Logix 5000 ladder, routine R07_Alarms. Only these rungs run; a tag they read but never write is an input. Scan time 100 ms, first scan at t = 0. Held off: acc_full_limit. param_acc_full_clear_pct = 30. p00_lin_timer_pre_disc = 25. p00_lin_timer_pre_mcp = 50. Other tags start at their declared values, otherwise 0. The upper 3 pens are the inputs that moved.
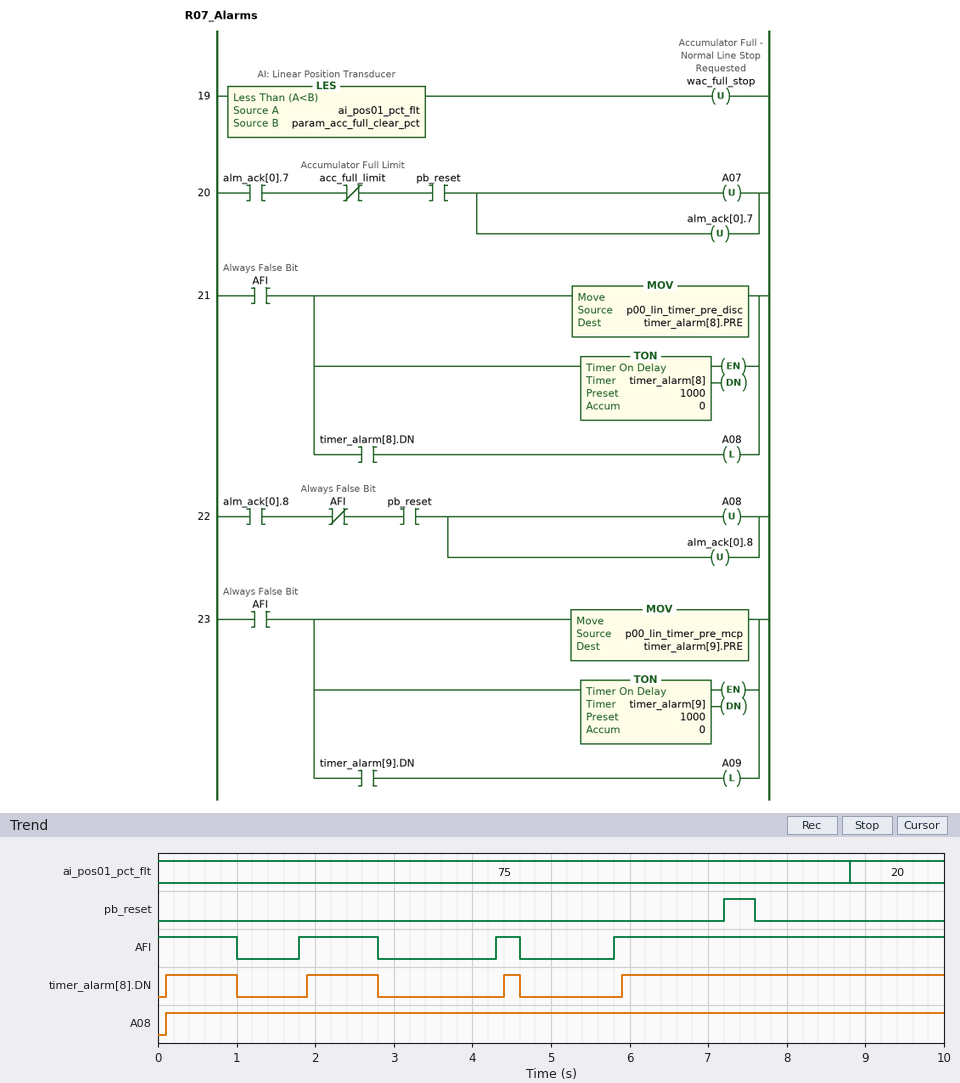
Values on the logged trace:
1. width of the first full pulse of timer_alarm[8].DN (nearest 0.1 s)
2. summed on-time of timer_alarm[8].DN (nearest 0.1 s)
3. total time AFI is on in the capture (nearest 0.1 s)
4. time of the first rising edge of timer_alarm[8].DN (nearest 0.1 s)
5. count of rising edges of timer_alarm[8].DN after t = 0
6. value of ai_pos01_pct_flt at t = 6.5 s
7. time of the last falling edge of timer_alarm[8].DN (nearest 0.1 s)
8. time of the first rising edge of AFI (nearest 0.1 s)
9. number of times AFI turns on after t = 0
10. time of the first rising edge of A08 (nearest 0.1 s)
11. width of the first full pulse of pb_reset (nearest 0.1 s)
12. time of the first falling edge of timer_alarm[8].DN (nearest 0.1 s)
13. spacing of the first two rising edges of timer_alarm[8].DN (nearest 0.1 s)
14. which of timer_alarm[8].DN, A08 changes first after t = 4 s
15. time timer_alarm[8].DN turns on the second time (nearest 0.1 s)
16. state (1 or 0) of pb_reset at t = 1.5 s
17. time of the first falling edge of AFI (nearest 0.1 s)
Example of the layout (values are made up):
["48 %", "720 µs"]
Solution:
["0.9 s", "6.1 s", "6.5 s", "0.1 s", "4", "75", "4.6 s", "1.8 s", "3", "0.1 s", "0.4 s", "1.0 s", "1.8 s", "timer_alarm[8].DN", "1.9 s", "0", "1.0 s"]
